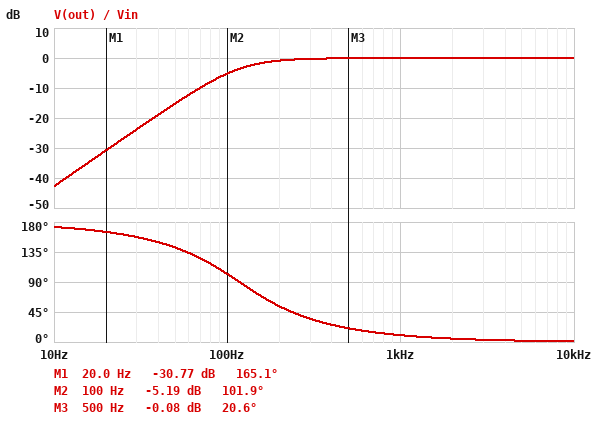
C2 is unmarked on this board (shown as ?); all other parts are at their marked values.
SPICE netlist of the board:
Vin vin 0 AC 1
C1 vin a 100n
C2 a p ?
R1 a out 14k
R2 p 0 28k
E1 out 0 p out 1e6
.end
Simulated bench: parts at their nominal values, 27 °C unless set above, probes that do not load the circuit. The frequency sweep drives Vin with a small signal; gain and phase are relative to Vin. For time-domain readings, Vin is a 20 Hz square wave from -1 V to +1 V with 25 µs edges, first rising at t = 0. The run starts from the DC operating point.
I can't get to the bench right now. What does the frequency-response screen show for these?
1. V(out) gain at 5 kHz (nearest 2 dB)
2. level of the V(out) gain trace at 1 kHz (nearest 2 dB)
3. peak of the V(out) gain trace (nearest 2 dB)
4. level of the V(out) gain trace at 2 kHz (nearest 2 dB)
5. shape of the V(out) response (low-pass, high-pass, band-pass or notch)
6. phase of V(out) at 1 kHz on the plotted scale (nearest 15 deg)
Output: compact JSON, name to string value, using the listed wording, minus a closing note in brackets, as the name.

{"V(out) gain at 5 kHz": "0 dB", "level of the V(out) gain trace at 1 kHz": "0 dB", "peak of the V(out) gain trace": "0 dB", "level of the V(out) gain trace at 2 kHz": "0 dB", "shape of the V(out) response": "high-pass", "phase of V(out) at 1 kHz on the plotted scale": "15 deg"}
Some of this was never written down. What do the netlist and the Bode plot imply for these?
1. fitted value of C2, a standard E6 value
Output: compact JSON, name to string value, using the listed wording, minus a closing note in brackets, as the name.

{"fitted value of C2, a standard E6 value": "47 nF"}
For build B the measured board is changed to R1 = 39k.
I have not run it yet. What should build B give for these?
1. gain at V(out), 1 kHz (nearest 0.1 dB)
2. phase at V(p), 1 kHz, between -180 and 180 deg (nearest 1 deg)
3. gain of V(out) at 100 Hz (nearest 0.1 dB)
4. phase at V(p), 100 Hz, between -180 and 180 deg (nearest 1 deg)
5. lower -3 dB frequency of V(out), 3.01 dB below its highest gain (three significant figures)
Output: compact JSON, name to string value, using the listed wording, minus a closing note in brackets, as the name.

{"gain at V(out), 1 kHz": "-0.1 dB", "phase at V(p), 1 kHz, between -180 and 180 deg": "10 deg", "gain of V(out) at 100 Hz": "-5.3 dB", "phase at V(p), 100 Hz, between -180 and 180 deg": "74 deg", "lower -3 dB frequency of V(out), 3.01 dB below its highest gain": "151 Hz"}
